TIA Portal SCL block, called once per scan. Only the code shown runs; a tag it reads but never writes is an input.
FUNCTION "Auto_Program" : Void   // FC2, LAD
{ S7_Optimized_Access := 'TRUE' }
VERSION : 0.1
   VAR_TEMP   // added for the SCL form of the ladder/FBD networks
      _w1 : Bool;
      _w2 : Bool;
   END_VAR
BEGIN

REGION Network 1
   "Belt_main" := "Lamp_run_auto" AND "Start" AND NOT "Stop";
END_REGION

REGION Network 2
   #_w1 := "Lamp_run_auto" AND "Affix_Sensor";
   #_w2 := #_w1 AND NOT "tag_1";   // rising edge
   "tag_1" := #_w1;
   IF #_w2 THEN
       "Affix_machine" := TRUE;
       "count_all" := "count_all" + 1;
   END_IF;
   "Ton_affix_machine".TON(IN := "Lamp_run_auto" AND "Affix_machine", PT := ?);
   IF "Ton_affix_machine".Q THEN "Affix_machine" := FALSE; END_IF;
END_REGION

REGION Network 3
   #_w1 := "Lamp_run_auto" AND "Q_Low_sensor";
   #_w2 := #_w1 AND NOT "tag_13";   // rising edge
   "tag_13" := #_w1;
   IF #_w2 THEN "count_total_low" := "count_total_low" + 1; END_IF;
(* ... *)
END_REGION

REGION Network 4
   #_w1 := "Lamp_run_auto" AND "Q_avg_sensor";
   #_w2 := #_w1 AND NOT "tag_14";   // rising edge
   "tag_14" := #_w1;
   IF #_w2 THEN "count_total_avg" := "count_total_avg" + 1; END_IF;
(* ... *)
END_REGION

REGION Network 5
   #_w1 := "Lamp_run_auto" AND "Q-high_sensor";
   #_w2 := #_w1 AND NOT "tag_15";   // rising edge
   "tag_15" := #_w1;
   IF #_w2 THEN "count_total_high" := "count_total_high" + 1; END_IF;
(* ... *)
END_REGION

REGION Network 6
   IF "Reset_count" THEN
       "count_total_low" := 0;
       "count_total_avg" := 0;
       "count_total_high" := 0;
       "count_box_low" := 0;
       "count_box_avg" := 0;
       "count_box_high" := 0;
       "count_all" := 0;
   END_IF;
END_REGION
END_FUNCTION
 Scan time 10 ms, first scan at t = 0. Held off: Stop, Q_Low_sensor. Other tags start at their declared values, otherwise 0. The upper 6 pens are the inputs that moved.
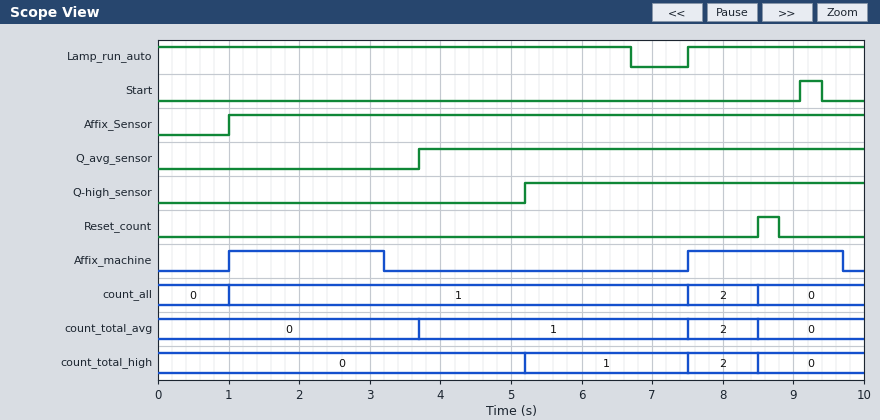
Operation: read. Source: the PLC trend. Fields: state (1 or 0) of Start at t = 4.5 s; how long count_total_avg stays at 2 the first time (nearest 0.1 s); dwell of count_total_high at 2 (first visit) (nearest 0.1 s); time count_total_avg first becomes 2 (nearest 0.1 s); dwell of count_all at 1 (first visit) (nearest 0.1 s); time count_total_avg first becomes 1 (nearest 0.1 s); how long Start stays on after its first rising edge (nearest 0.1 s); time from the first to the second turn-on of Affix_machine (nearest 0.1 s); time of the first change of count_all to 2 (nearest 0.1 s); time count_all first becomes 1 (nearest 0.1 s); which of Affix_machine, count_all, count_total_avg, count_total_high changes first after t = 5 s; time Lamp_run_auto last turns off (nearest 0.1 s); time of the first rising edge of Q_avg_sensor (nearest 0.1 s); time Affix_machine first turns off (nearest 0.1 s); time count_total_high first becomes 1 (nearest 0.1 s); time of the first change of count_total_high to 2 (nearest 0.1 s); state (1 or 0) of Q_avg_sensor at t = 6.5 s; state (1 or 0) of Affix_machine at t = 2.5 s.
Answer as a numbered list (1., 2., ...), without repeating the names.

1. 0
2. 1.0 s
3. 1.0 s
4. 7.5 s
5. 6.5 s
6. 3.7 s
7. 0.3 s
8. 6.5 s
9. 7.5 s
10. 1.0 s
11. count_total_high
12. 6.7 s
13. 3.7 s
14. 3.2 s
15. 5.2 s
16. 7.5 s
17. 1
18. 1
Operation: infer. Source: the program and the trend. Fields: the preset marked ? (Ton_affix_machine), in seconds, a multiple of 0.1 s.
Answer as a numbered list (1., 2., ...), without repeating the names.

1. 2.2 s
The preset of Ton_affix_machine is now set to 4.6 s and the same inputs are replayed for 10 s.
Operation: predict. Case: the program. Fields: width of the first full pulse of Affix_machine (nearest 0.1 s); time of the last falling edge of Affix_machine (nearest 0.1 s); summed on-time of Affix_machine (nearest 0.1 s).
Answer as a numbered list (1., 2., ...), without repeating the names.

1. 4.6 s
2. 5.6 s
3. 7.1 s
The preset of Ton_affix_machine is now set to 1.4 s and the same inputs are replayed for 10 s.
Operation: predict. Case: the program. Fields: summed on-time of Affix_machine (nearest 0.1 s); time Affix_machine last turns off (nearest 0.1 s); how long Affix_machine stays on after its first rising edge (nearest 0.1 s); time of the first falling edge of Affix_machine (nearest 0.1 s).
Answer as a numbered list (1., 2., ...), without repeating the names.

1. 2.8 s
2. 8.9 s
3. 1.4 s
4. 2.4 s
